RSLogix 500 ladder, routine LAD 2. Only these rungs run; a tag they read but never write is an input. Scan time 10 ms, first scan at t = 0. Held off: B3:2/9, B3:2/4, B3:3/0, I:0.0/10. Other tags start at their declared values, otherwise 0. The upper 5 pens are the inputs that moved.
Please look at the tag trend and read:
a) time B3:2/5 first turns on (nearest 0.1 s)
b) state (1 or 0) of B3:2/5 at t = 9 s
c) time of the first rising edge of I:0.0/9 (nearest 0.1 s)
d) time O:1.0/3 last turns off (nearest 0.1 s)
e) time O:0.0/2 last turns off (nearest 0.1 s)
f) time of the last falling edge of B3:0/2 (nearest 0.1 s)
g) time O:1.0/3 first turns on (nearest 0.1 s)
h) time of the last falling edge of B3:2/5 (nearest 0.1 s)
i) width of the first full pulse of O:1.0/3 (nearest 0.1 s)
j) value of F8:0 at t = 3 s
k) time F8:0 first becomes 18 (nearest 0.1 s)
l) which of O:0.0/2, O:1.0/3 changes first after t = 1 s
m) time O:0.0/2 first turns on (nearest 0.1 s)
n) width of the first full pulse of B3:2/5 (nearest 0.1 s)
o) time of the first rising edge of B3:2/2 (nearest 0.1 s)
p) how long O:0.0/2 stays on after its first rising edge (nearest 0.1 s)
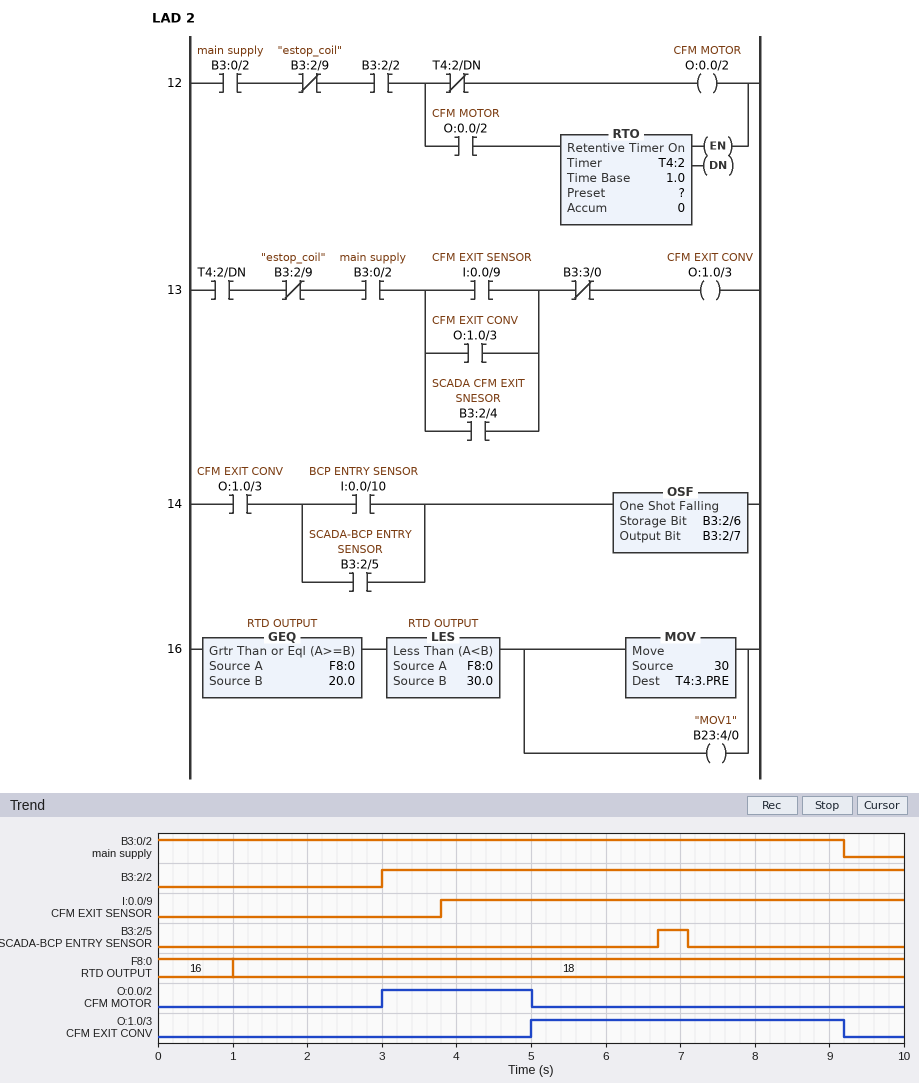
6.7 s
0
3.8 s
9.2 s
5.0 s
9.2 s
5.0 s
7.1 s
4.2 s
18
1.0 s
O:0.0/2
3.0 s
0.4 s
3.0 s
2.0 s
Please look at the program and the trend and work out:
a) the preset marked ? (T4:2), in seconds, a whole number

2 s
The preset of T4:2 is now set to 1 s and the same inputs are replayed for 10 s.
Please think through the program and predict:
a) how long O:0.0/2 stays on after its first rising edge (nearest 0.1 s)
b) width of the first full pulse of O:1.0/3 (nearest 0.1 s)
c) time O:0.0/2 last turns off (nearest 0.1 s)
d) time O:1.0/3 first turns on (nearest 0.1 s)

1.0 s
5.2 s
4.0 s
4.0 s
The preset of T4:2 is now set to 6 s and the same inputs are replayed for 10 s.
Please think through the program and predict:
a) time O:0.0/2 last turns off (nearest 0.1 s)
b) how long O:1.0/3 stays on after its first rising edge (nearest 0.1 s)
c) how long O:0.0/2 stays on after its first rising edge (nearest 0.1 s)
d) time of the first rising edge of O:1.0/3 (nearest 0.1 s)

9.0 s
0.2 s
6.0 s
9.0 s
